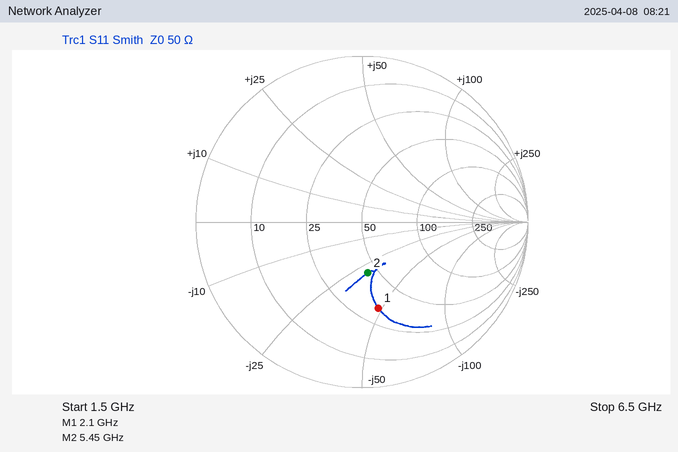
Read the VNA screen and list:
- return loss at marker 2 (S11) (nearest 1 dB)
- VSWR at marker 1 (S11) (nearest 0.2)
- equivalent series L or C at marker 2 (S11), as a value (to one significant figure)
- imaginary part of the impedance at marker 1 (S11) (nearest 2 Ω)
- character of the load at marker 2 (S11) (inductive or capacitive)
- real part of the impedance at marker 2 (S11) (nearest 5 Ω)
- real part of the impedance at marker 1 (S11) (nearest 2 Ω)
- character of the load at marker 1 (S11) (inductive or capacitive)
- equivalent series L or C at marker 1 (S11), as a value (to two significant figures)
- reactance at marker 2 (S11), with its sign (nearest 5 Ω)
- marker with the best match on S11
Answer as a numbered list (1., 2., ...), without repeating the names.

1. 10 dB
2. 3.2
3. 1.0 pF
4. -48 Ω
5. capacitive
6. 45 Ω
7. 34 Ω
8. capacitive
9. 1.6 pF
10. -30 Ω
11. marker 2
